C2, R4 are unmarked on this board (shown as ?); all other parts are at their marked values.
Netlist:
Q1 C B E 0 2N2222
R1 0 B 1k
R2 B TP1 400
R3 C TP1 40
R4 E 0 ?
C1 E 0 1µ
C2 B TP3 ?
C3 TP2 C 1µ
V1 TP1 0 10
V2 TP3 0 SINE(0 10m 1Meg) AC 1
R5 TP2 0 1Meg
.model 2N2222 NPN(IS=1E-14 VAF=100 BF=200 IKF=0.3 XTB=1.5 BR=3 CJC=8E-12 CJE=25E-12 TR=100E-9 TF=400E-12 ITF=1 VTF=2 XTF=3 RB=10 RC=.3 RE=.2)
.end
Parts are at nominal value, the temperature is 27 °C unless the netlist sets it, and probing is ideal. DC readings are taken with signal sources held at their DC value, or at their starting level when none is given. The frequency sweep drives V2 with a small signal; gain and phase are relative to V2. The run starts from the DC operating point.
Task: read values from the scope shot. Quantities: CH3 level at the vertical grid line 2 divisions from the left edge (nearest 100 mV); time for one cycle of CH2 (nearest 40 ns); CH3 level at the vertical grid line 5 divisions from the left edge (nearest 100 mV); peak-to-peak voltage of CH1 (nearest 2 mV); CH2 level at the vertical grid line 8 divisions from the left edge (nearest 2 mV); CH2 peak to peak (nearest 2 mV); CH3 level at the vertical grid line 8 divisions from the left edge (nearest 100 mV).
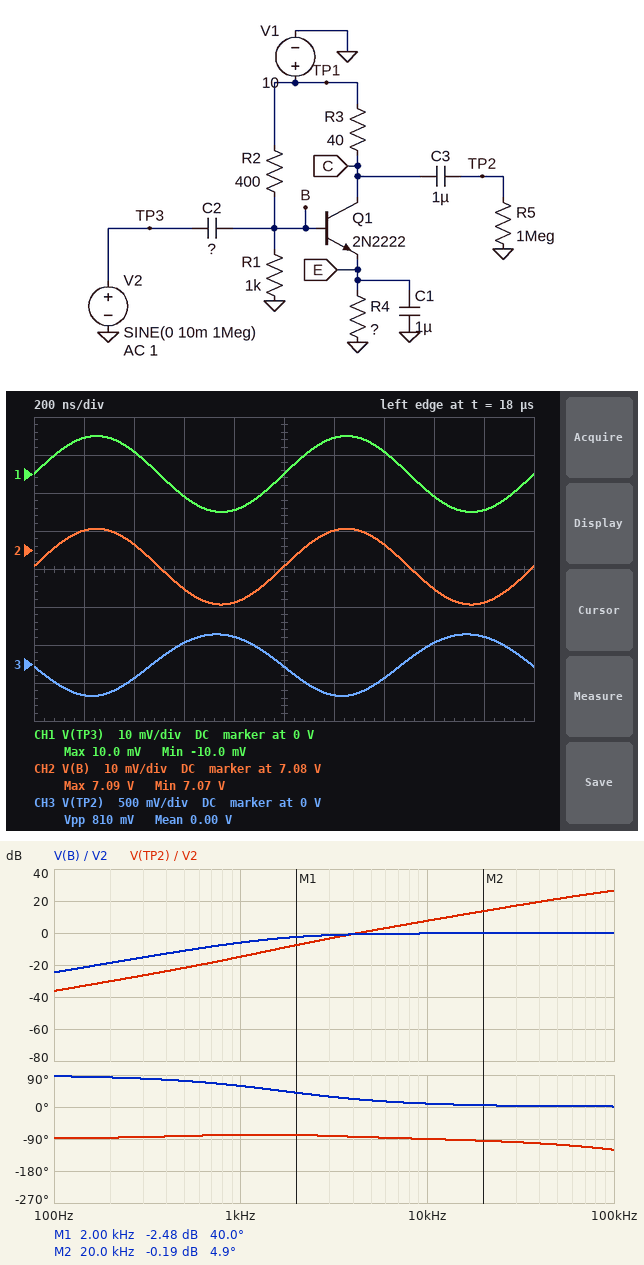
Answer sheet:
-200 mV
1.00 µs
0 V
20 mV
7.070 V
20 mV
300 mV
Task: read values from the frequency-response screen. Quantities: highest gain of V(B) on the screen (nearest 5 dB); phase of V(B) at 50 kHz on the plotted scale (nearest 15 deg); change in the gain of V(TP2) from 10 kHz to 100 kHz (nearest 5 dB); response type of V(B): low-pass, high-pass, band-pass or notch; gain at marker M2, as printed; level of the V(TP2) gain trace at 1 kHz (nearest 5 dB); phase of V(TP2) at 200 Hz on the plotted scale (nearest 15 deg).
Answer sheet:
0 dB
0 deg
20 dB
high-pass
-0.19 dB
-15 dB
-90 deg
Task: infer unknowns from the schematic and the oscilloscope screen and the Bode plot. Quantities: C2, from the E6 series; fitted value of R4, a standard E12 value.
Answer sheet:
330 nF
150 Ω
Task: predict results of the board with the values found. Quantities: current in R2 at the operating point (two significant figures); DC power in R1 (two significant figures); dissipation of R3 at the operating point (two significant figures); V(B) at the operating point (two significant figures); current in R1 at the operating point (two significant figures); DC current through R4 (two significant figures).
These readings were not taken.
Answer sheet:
7.3 mA
50 mW
70 mW
7.1 V
7.1 mA
42 mA
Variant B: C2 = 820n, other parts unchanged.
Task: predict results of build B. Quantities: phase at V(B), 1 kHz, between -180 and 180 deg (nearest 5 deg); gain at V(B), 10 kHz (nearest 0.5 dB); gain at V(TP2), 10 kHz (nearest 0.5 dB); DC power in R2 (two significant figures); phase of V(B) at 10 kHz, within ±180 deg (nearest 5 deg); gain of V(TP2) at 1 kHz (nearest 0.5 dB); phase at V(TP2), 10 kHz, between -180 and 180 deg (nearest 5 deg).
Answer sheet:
35 deg
0 dB
8.0 dB
21 mW
5 deg
-10.5 dB
-95 deg
